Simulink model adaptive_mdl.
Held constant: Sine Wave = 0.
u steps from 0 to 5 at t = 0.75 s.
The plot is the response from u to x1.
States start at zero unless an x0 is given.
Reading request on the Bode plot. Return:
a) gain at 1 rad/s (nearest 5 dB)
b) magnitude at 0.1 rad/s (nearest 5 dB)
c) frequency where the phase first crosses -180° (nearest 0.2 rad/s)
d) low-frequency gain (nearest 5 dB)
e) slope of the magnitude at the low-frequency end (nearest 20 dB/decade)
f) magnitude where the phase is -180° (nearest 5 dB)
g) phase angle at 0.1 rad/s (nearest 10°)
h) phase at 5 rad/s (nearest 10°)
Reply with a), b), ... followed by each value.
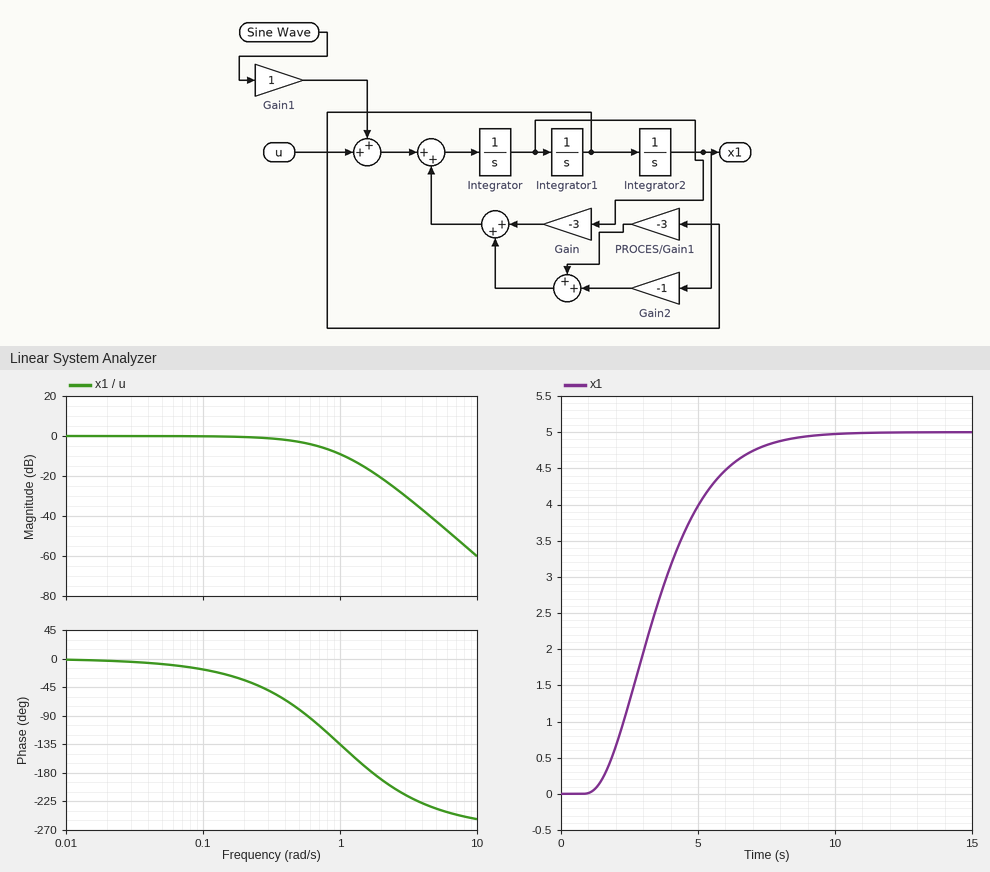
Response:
a) -10 dB
b) 0 dB
c) 1.8 rad/s
d) 0 dB
e) 0 dB/decade
f) -20 dB
g) -20°
h) -240°
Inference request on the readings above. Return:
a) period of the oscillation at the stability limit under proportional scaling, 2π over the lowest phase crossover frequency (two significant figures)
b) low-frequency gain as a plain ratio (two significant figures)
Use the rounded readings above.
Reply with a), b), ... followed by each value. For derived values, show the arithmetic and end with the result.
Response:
a) 2π / 1.8 = 3.5 s
b) 10^(0 / 20) = 1.0
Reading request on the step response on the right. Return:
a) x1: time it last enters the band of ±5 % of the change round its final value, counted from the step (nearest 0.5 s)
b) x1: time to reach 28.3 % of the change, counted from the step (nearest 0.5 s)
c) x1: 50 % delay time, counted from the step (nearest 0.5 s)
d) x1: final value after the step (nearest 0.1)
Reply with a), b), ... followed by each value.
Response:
a) 6.5 s
b) 2.0 s
c) 2.5 s
d) 5.0
